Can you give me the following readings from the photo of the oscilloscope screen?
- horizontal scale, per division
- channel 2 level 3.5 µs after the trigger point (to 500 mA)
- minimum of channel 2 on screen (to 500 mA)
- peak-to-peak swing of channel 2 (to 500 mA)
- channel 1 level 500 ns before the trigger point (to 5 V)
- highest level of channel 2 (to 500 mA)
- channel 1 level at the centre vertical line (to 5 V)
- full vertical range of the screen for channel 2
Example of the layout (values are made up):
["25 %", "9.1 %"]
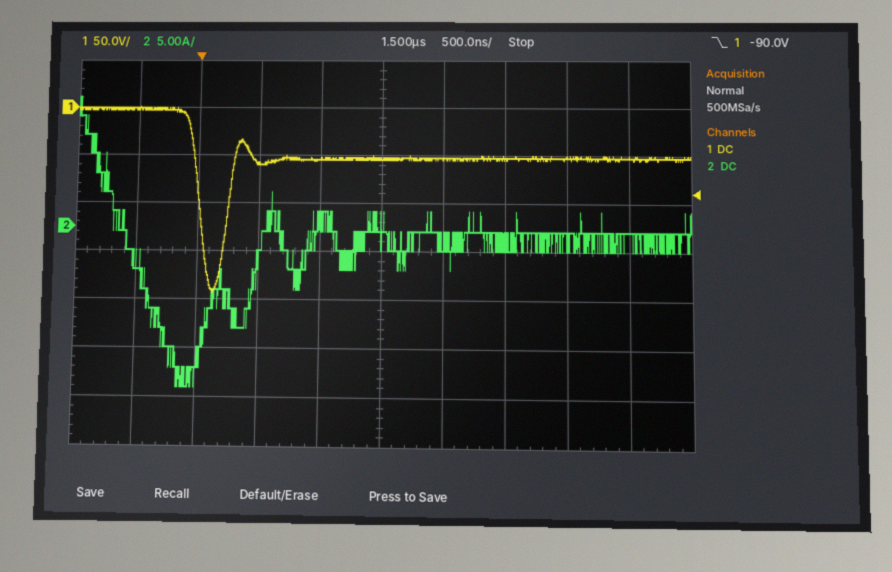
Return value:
["500 ns", "-500 mA", "-16.5 A", "30.0 A", "0 V", "13.5 A", "-55 V", "40 A"]
